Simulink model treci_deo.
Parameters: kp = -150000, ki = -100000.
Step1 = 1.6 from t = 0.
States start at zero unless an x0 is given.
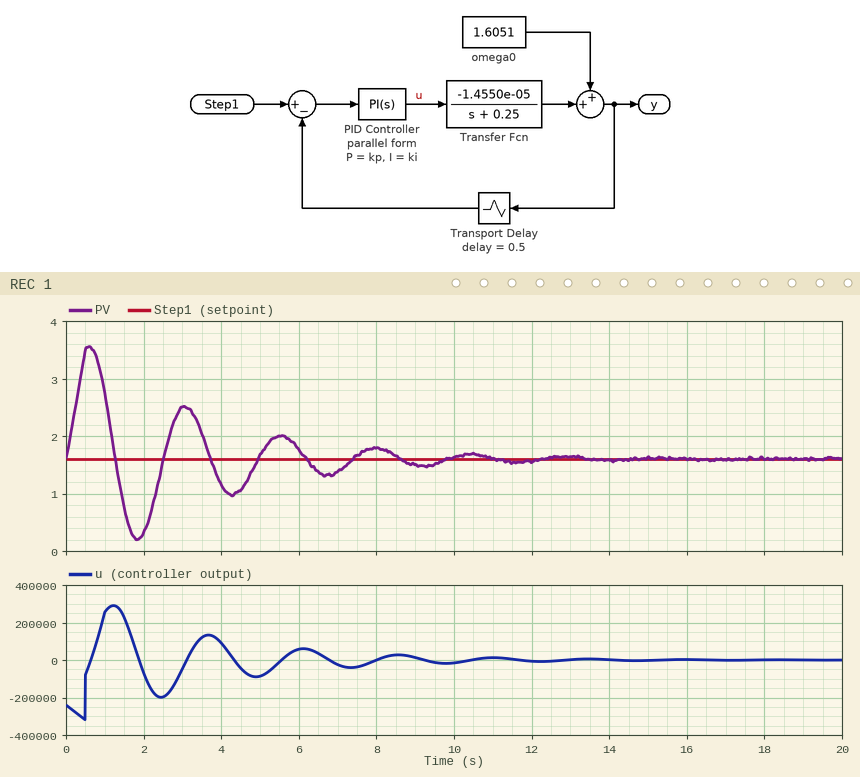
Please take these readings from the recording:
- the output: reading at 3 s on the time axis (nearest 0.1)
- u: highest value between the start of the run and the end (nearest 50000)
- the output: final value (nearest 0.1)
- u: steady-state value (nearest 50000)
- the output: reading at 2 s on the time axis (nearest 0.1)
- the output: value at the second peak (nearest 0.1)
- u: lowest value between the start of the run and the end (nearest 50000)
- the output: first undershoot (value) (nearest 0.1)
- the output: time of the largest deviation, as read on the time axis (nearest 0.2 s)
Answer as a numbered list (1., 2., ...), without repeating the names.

1. 2.5
2. 300000
3. 1.6
4. 0
5. 0.3
6. 2.5
7. -300000
8. 0.2
9. 0.6 s
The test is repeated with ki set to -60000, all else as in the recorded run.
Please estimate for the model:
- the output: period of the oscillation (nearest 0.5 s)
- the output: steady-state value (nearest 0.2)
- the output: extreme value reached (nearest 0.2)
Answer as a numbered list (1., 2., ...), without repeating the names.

1. 2.5 s
2. 1.6
3. 3.4
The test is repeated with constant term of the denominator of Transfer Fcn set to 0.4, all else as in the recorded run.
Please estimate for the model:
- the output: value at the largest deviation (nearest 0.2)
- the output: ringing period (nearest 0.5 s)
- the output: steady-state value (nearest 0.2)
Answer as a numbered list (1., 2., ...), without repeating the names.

1. 3.4
2. 2.5 s
3. 1.6
